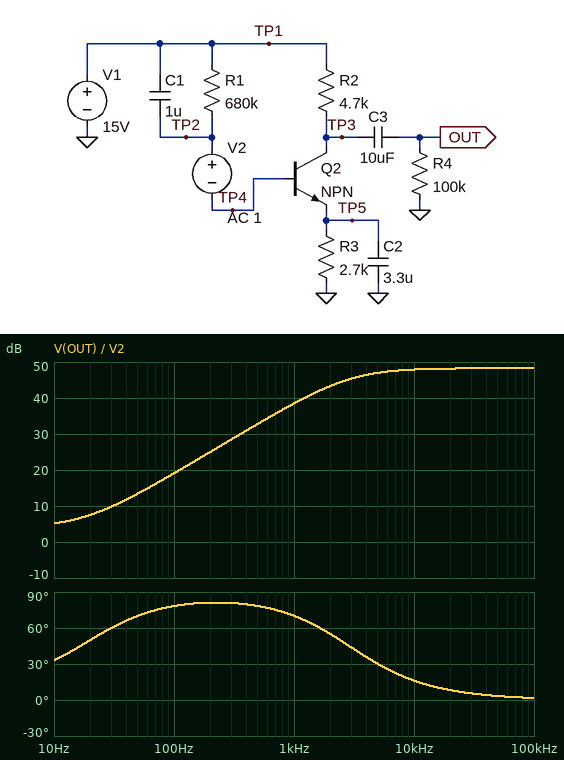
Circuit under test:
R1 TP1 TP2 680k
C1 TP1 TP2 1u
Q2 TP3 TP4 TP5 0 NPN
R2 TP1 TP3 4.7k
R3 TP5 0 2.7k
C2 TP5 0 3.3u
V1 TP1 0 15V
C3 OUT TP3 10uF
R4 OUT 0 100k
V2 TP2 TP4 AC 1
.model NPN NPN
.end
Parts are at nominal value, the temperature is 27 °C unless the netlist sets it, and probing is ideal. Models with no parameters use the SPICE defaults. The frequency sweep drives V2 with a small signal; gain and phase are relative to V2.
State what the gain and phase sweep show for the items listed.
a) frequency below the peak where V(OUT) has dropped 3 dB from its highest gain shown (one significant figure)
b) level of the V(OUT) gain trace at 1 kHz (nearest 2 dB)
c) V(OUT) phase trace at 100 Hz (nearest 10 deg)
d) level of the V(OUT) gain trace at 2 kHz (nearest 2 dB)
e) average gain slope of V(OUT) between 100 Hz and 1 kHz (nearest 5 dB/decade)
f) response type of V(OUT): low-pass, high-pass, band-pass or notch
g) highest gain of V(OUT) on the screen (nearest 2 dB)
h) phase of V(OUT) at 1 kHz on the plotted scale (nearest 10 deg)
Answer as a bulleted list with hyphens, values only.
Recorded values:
- 3 kHz
- 38 dB
- 80 deg
- 44 dB
- 20 dB/decade
- high-pass
- 48 dB
- 70 deg
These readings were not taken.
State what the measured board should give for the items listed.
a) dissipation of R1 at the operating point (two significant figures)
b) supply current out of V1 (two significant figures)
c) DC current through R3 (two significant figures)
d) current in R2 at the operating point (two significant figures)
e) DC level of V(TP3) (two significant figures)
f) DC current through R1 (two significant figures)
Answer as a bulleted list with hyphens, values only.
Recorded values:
- 150 µW
- 1.5 mA
- 1.5 mA
- 1.5 mA
- 8.0 V
- 15 µA
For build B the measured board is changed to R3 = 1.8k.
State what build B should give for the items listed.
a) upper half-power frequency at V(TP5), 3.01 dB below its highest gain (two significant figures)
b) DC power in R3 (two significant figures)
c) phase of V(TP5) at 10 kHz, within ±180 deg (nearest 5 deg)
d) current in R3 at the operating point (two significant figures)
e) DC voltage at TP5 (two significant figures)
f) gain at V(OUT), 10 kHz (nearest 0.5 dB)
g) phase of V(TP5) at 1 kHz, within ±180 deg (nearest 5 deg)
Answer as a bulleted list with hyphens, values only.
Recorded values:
- 3.2 kHz
- 5.0 mW
- 110 deg
- 1.7 mA
- 3.0 V
- 48.5 dB
- 165 deg
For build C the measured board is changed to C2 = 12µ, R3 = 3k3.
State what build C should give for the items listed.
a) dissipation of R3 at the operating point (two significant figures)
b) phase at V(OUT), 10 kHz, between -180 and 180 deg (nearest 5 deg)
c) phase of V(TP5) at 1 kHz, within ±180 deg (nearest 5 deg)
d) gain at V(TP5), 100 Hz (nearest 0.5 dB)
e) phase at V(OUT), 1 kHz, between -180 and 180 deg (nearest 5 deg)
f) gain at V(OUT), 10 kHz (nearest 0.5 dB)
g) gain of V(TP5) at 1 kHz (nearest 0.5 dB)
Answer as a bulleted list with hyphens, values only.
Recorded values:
- 6.6 mW
- 5 deg
- 130 deg
- -1.0 dB
- 40 deg
- 47.5 dB
- -5.0 dB
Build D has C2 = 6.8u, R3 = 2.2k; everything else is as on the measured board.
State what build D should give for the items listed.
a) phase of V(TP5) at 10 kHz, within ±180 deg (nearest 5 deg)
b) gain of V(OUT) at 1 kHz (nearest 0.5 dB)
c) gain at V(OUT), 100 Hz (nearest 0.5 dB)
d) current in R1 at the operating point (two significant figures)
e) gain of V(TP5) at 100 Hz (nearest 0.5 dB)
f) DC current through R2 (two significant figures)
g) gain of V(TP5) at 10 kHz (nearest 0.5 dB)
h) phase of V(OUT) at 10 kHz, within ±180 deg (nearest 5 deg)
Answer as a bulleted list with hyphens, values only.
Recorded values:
- 100 deg
- 43.5 dB
- 25.0 dB
- 16 µA
- -0.5 dB
- 1.6 mA
- -17.0 dB
- 10 deg
